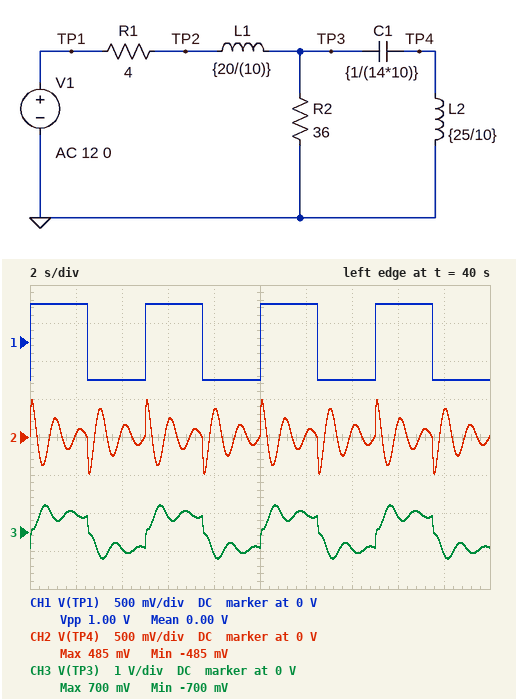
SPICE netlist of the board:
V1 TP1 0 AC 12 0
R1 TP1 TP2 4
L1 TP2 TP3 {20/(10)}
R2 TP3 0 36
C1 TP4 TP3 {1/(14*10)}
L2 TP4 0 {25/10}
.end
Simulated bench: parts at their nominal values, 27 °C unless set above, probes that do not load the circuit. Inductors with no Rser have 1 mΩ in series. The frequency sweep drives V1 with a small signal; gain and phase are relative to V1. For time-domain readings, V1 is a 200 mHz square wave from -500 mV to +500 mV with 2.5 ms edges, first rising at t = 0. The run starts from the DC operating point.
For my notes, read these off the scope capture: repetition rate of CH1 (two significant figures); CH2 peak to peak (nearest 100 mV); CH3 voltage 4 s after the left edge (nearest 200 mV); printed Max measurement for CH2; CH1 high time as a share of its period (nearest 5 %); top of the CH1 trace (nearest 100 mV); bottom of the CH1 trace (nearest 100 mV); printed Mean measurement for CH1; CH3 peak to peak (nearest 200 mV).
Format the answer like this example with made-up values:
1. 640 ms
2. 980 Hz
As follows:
1. 200 mHz
2. 1.0 V
3. -400 mV
4. 485 mV
5. 50 %
6. 500 mV
7. -500 mV
8. 0.00 V
9. 1.4 V
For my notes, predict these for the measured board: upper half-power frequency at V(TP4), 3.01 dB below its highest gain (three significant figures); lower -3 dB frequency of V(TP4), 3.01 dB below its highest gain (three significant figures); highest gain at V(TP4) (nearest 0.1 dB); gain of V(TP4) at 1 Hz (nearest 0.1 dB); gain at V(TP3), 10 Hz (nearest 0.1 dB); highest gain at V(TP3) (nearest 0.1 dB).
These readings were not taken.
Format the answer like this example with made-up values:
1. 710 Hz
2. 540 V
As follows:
1. 1.11 Hz
2. 838 mHz
3. 6.3 dB
4. 5.6 dB
5. -12.0 dB
6. 3.5 dB
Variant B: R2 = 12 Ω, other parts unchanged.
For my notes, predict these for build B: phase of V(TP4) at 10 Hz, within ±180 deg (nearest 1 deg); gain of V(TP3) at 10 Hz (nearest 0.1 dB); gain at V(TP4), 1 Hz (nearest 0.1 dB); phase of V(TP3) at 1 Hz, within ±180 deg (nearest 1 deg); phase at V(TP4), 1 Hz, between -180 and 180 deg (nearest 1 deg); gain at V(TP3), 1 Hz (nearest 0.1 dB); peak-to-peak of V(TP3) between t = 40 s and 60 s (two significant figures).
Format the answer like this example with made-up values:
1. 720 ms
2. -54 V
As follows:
1. -78 deg
2. -20.6 dB
3. 2.7 dB
4. -109 deg
5. 71 deg
6. -4.9 dB
7. 1.0 V
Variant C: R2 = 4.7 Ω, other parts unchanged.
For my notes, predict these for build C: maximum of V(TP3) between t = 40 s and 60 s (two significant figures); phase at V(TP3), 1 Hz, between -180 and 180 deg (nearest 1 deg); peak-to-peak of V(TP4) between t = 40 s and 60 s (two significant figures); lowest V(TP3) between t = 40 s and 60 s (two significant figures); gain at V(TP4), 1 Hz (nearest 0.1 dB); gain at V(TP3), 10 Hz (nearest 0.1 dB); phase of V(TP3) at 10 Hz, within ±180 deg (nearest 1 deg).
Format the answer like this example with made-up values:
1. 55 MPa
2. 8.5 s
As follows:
1. 290 mV
2. -91 deg
3. 370 mV
4. -290 mV
5. -2.8 dB
6. -28.6 dB
7. -84 deg
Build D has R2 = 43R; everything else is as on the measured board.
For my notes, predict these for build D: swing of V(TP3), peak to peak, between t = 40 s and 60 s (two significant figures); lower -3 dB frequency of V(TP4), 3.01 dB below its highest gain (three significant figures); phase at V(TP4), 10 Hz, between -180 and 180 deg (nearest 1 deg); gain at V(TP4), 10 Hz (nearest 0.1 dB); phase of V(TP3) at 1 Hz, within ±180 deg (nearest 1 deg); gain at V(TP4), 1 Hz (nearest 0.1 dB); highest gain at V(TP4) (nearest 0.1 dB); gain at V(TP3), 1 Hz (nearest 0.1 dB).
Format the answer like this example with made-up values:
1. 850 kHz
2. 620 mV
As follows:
1. 1.4 V
2. 835 mHz
3. -57 deg
4. -10.7 dB
5. -132 deg
6. 5.9 dB
7. 6.8 dB
8. -1.7 dB
